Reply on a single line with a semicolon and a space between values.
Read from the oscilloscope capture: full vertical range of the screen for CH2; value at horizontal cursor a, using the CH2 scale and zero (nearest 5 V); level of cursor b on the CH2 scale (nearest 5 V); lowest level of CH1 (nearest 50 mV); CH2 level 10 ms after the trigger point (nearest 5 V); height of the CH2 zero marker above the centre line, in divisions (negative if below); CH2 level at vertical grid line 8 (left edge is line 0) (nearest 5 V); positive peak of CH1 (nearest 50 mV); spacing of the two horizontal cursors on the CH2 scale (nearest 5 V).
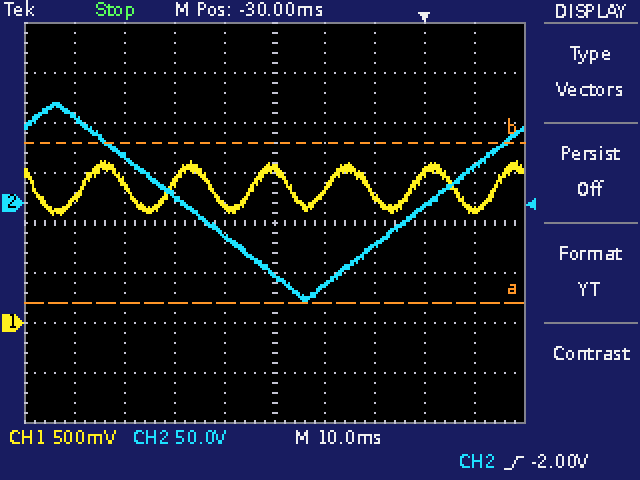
400 V; -100 V; 60 V; 1.10 V; 35 V; +0.4 div; -5 V; 1.60 V; 160 V
